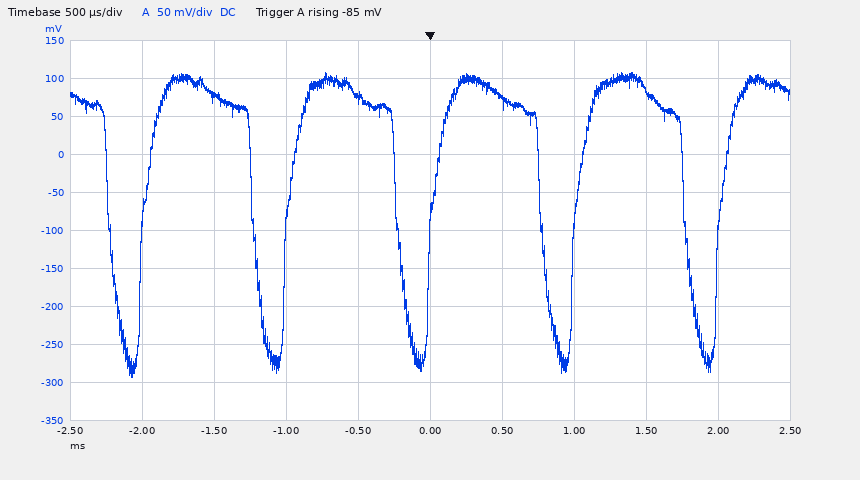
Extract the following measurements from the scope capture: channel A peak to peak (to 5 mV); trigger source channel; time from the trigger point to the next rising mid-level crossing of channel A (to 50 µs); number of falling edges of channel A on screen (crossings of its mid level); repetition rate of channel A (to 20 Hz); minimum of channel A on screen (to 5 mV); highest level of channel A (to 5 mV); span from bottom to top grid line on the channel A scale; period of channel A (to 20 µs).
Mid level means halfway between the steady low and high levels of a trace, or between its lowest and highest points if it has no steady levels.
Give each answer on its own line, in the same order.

400 mV
channel A
1.00 ms
5
1.00 kHz
-290 mV
110 mV
500 mV
1.00 ms
